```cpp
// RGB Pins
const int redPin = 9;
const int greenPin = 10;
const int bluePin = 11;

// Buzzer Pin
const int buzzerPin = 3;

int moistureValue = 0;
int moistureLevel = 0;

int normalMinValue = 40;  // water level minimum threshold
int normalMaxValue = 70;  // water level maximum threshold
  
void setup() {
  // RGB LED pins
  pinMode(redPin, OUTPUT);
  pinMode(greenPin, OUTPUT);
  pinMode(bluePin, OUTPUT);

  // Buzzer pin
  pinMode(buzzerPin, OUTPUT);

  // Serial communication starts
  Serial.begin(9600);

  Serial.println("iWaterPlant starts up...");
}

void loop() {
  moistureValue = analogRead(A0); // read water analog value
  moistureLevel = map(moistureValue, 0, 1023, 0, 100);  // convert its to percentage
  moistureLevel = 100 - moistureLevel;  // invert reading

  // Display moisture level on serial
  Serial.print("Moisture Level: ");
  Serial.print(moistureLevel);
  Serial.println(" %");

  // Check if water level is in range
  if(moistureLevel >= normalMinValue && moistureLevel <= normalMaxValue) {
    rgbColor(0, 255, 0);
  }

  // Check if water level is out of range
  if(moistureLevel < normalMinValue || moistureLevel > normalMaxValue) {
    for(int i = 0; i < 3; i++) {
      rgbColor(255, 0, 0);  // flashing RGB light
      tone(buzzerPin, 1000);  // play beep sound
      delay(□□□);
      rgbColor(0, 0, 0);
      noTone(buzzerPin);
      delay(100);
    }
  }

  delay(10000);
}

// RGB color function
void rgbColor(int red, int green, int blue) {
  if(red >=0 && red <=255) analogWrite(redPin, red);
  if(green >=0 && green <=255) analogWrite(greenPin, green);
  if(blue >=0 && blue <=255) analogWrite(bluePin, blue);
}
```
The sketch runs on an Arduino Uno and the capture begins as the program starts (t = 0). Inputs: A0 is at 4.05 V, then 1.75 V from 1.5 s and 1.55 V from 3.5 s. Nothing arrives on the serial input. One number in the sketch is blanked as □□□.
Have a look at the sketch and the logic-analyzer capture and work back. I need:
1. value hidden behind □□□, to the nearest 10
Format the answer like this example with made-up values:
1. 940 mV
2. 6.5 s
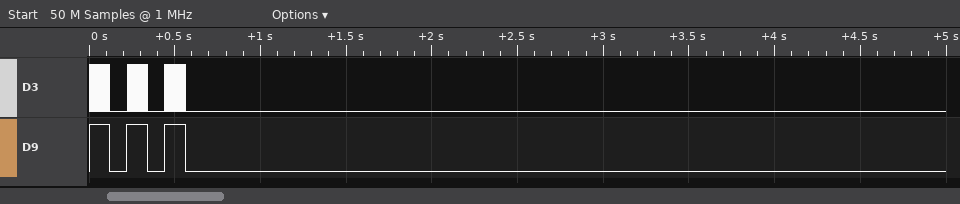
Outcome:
1. 120
